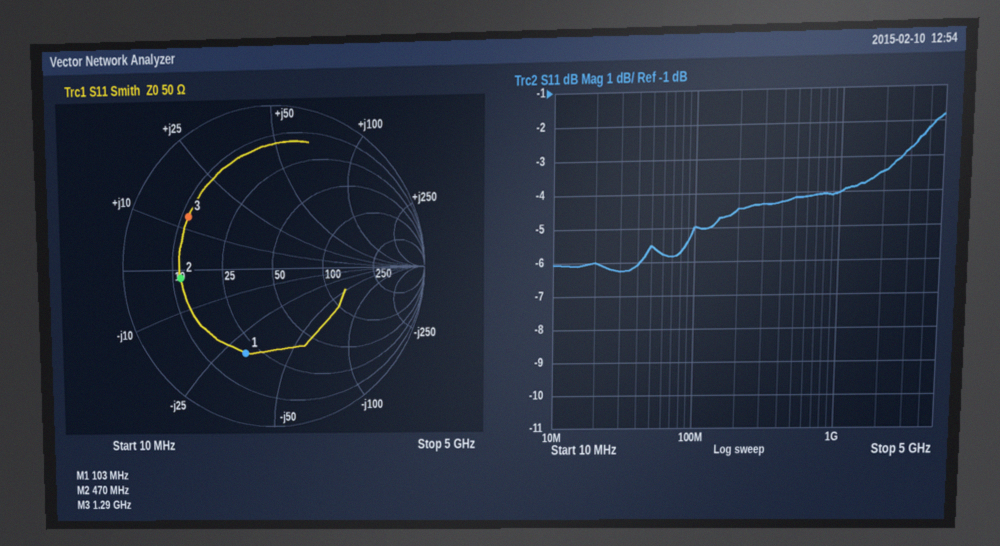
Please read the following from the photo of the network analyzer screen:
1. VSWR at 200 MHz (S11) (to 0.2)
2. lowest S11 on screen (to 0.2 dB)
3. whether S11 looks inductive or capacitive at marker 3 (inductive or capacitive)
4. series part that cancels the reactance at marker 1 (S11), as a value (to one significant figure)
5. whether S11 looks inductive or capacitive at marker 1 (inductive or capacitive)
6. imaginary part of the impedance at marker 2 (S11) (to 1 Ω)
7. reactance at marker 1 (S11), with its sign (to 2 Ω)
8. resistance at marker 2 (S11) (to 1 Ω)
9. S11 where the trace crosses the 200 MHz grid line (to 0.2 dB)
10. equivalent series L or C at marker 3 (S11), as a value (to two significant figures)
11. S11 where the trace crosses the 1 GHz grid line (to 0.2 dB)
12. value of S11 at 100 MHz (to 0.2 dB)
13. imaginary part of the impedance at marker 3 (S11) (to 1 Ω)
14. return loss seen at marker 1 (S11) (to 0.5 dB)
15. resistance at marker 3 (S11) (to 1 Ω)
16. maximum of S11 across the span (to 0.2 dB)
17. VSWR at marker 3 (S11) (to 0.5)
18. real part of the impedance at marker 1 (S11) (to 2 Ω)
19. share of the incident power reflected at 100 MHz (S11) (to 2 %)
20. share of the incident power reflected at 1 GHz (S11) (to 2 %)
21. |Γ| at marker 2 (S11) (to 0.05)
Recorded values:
4.0
-6.2 dB
inductive
50 nH
capacitive
-2 Ω
-32 Ω
12 Ω
-4.4 dB
1.6 nH
-4.0 dB
-5.0 dB
+13 Ω
5.0 dB
12 Ω
-1.8 dB
4.5
20 Ω
32 %
40 %
0.60
